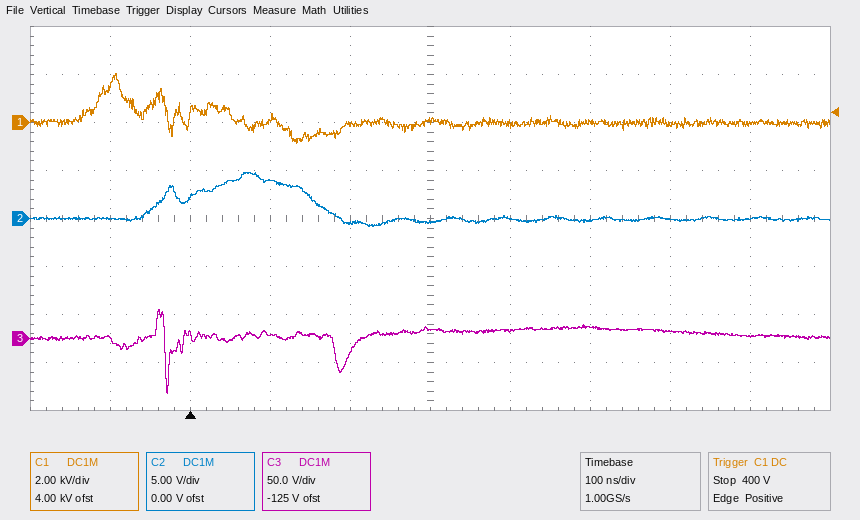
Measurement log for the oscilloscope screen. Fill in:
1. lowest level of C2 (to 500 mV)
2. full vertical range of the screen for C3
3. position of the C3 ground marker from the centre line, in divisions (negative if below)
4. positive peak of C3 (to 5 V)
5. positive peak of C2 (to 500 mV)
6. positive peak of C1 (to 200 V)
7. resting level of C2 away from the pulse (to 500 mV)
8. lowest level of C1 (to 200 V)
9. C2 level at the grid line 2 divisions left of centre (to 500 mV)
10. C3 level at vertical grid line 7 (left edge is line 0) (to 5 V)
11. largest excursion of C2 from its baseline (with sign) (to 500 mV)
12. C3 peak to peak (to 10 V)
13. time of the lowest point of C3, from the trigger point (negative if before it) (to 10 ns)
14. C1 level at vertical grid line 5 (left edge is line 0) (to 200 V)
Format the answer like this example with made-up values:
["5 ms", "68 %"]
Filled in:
["-1.0 V", "400 V", "-2.5 div", "30 V", "5.0 V", "2.0 kV", "0.0 V", "-800 V", "4.0 V", "10 V", "+5.0 V", "90 V", "-30 ns", "0.0 kV"]
